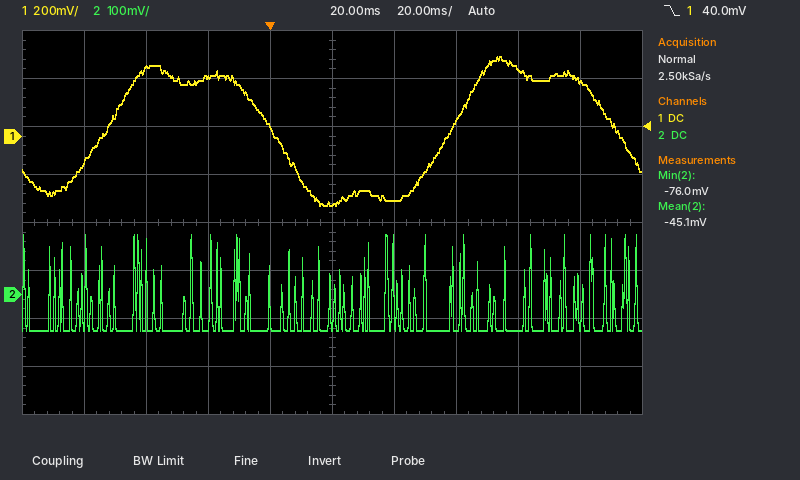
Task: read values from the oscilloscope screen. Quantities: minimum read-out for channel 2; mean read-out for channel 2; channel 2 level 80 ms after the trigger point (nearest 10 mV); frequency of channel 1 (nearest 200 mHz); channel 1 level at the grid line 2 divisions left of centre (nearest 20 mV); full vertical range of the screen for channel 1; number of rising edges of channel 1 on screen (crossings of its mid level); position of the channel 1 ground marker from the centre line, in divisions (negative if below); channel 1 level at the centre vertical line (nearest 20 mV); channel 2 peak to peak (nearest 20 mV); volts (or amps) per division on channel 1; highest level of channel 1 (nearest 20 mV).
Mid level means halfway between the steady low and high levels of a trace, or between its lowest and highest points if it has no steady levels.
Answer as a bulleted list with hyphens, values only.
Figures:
- -76.0 mV
- -45.1 mV
- -80 mV
- 9.0 Hz
- 240 mV
- 1.6 V
- 2
- +1.8 div
- -280 mV
- 200 mV
- 200 mV
- 340 mV
